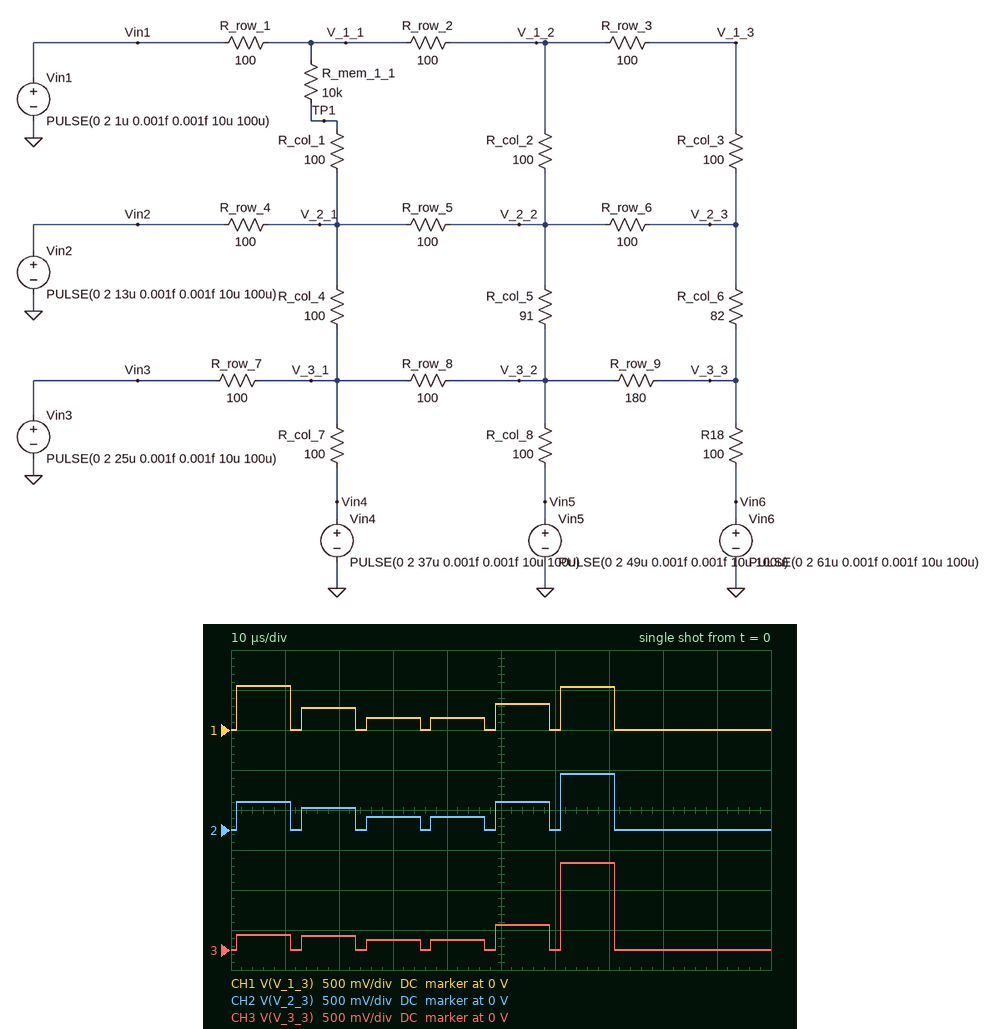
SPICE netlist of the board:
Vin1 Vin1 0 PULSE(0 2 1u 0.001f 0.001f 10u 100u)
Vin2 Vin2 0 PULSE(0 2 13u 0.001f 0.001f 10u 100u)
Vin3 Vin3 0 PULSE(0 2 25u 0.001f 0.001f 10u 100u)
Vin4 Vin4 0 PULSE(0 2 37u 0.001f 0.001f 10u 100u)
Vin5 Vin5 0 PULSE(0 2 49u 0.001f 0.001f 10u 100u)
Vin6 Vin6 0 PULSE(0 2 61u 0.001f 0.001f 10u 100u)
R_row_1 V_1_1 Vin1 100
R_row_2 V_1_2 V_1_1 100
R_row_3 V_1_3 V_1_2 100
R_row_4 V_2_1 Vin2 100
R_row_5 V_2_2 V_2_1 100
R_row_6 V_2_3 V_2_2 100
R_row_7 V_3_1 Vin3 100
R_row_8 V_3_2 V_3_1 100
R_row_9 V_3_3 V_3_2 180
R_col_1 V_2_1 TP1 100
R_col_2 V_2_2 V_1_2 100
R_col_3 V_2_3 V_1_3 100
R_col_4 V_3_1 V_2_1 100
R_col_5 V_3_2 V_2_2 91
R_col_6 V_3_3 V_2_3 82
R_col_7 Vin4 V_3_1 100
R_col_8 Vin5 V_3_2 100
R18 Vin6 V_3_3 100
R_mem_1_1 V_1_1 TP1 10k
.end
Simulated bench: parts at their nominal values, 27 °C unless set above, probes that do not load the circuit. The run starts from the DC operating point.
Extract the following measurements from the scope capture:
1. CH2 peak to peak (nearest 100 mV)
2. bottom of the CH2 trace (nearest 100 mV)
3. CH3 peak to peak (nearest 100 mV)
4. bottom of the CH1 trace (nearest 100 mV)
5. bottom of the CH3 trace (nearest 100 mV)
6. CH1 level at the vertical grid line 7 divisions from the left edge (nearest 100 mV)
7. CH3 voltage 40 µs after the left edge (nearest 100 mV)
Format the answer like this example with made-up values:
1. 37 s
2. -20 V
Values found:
1. 700 mV
2. 0 V
3. 1.1 V
4. 0 V
5. 0 V
6. 500 mV
7. 100 mV
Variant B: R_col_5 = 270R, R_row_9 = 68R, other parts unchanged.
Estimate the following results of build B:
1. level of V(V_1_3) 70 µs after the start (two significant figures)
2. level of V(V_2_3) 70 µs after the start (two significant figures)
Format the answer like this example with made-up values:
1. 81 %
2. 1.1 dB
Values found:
1. 480 mV
2. 620 mV
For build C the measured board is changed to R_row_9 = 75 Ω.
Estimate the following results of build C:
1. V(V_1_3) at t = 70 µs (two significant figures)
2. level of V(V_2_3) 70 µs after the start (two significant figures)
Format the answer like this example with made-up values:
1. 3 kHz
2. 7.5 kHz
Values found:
1. 490 mV
2. 630 mV
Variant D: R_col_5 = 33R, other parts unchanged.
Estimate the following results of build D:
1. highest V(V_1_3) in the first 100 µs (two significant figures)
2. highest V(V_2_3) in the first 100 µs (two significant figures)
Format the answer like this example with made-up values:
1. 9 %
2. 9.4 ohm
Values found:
1. 520 mV
2. 690 mV
